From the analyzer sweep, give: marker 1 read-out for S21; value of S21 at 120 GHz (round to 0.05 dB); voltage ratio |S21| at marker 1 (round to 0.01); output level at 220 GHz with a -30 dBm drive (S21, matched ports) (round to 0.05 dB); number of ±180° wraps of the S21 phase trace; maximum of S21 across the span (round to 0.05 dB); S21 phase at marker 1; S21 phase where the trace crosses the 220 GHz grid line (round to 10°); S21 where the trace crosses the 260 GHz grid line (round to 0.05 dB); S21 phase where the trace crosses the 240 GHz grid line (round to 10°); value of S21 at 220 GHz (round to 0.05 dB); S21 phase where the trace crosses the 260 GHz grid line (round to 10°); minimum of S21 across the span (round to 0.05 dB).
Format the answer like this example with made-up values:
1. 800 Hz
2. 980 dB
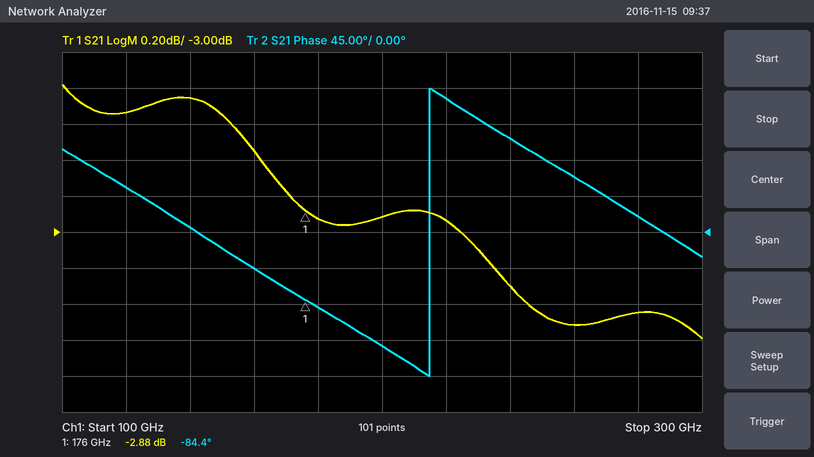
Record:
1. -2.88 dB
2. -2.35 dB
3. 0.72
4. -32.95 dBm
5. 1
6. -2.20 dB
7. -84.4°
8. 170°
9. -3.50 dB
10. 120°
11. -2.95 dB
12. 70°
13. -3.60 dB
